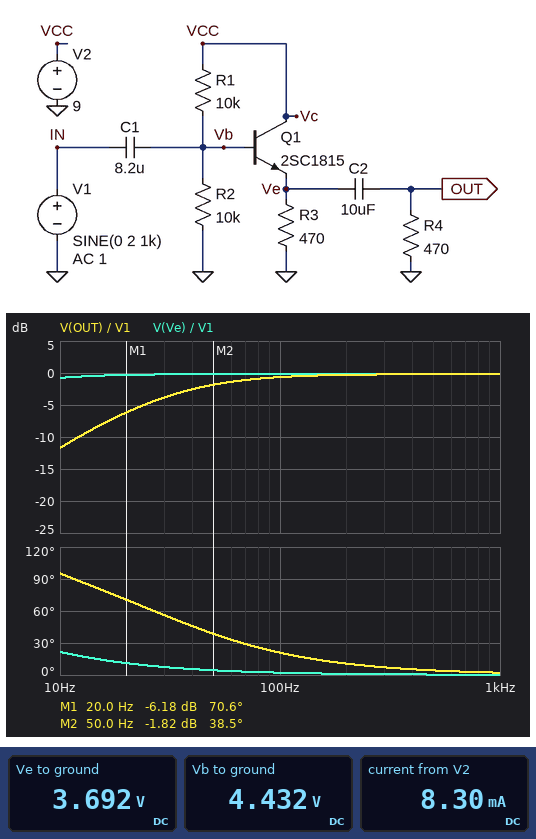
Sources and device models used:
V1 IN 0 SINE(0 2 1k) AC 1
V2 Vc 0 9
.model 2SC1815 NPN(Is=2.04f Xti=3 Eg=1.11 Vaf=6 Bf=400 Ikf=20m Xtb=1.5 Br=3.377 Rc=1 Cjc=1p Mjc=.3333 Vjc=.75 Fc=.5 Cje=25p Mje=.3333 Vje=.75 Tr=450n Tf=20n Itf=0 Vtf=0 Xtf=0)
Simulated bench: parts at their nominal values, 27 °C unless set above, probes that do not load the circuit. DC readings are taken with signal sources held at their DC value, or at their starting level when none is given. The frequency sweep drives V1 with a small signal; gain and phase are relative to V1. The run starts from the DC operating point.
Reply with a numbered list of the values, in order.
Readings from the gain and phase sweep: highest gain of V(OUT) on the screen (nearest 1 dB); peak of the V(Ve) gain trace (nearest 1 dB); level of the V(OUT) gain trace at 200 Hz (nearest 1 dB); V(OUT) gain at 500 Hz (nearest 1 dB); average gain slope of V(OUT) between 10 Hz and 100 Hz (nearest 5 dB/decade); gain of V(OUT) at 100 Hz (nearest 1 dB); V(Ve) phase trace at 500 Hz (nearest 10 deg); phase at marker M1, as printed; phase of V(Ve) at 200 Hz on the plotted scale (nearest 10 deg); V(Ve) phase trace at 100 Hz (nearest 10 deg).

1. 0 dB
2. 0 dB
3. 0 dB
4. 0 dB
5. 10 dB/decade
6. -1 dB
7. 0 deg
8. 70.6 deg
9. 0 deg
10. 0 deg
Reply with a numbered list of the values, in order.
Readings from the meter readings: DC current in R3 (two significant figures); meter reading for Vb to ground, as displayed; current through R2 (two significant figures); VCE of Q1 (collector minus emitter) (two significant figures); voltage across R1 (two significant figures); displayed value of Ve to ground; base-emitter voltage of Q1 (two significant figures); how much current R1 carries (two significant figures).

1. 7.9 mA
2. 4.432 V
3. 440 µA
4. 5.3 V
5. 4.6 V
6. 3.692 V
7. 740 mV
8. 460 µA
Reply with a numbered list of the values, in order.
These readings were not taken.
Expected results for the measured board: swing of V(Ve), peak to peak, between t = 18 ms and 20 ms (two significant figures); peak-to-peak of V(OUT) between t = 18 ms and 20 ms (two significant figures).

1. 3.8 V
2. 3.8 V
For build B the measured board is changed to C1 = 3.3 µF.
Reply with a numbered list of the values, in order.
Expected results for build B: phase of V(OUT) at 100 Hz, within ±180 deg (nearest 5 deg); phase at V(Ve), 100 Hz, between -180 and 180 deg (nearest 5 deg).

1. 25 deg
2. 5 deg
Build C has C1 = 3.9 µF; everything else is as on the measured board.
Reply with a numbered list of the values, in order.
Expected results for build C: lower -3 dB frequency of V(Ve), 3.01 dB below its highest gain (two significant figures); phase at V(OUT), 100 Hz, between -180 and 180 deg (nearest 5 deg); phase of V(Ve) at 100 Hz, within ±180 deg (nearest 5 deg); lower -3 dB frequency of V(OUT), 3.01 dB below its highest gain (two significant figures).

1. 8.3 Hz
2. 25 deg
3. 5 deg
4. 36 Hz
